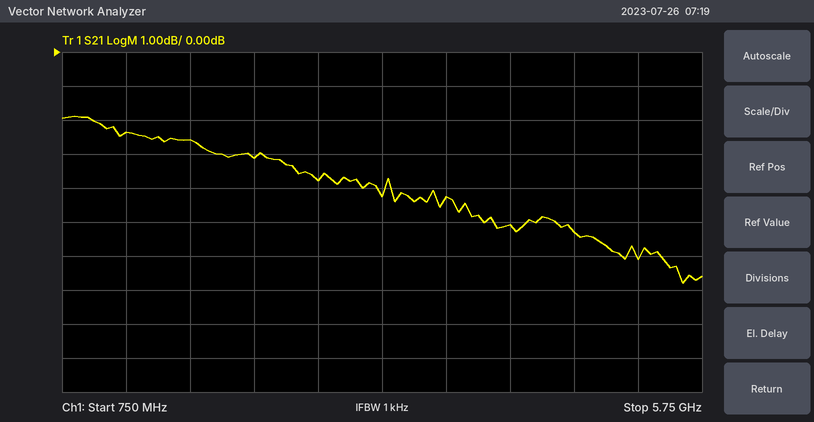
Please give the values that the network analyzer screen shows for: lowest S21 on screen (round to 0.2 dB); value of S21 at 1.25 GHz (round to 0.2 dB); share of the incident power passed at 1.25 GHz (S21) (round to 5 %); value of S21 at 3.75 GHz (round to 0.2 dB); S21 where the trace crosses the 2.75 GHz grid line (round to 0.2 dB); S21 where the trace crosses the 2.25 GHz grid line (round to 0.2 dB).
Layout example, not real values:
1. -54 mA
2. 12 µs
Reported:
1. -6.8 dB
2. -2.4 dB
3. 60 %
4. -4.2 dB
5. -3.8 dB
6. -3.2 dB
